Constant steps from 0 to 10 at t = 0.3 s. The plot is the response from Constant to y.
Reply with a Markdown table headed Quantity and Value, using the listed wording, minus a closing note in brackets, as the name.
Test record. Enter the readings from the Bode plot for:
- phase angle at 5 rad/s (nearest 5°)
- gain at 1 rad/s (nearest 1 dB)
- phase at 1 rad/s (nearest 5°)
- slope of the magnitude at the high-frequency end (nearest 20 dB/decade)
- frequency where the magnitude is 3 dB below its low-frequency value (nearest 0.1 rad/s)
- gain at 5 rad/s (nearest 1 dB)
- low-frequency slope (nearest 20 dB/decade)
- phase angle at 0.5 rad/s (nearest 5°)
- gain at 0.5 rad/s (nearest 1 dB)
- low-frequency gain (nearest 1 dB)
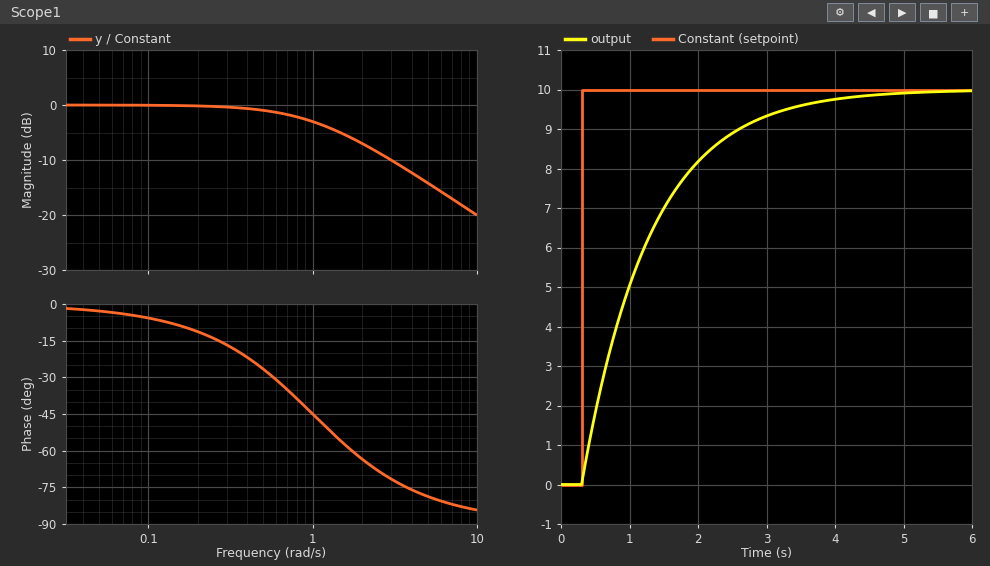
| Quantity | Value |
|---|---|
| phase angle at 5 rad/s | -80° |
| gain at 1 rad/s | -3 dB |
| phase at 1 rad/s | -45° |
| slope of the magnitude at the high-frequency end | -20 dB/decade |
| frequency where the magnitude is 3 dB below its low-frequency value | 1.0 rad/s |
| gain at 5 rad/s | -14 dB |
| low-frequency slope | 0 dB/decade |
| phase angle at 0.5 rad/s | -25° |
| gain at 0.5 rad/s | -1 dB |
| low-frequency gain | 0 dB |
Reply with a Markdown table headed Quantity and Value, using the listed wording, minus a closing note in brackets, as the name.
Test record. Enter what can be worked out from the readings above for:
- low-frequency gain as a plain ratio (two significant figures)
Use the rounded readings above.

| Quantity | Value |
|---|---|
| low-frequency gain as a plain ratio | 1.0 |
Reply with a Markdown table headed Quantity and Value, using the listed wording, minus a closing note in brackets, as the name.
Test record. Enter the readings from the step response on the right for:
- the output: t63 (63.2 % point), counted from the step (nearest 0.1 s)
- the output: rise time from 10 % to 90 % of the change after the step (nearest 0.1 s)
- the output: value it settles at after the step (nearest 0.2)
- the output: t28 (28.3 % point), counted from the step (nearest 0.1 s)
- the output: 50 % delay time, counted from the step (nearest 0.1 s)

| Quantity | Value |
|---|---|
| the output: t63 (63.2 % point), counted from the step | 1.0 s |
| the output: rise time from 10 % to 90 % of the change after the step | 2.2 s |
| the output: value it settles at after the step | 10.0 |
| the output: t28 (28.3 % point), counted from the step | 0.3 s |
| the output: 50 % delay time, counted from the step | 0.7 s |
